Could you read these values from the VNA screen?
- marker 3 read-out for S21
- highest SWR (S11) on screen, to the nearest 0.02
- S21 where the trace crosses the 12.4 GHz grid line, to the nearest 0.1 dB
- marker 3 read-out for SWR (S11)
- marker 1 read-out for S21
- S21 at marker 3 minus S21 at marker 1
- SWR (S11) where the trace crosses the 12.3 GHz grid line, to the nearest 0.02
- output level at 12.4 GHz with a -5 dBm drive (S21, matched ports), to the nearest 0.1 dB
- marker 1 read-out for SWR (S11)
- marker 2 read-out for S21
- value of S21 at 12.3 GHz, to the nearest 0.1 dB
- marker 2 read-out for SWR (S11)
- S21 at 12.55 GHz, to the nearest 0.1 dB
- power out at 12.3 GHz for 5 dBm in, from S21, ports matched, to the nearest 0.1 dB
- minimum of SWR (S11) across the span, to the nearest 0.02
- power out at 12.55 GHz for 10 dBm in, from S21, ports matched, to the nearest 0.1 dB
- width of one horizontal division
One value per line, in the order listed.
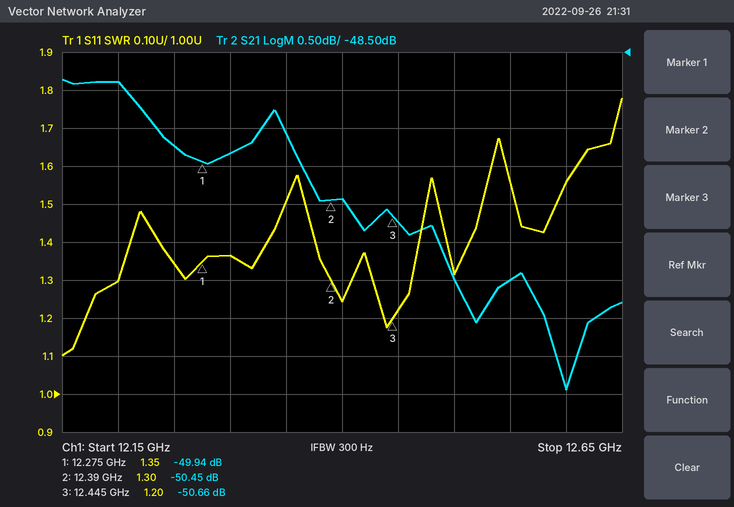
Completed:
-50.66 dB
1.78
-50.4 dB
1.20
-49.94 dB
-0.72 dB
1.36
-55.4 dBm
1.35
-50.45 dB
-49.8 dB
1.30
-51.5 dB
-44.8 dBm
1.10
-41.5 dBm
50 MHz
